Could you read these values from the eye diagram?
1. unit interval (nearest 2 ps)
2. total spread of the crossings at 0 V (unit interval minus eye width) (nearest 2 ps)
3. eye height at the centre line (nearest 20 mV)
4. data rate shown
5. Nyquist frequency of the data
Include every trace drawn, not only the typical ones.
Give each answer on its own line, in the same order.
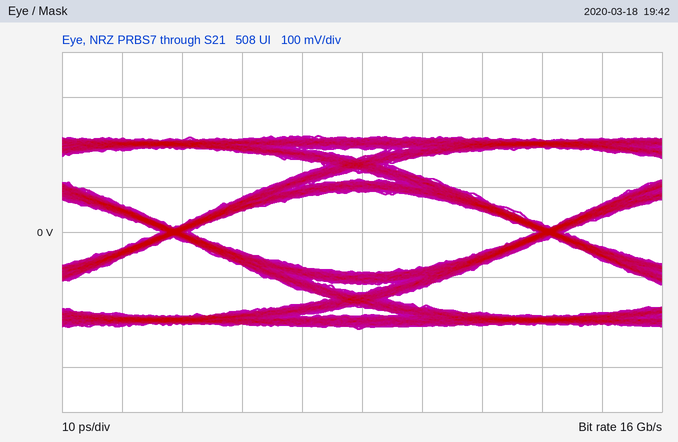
62 ps
4 ps
180 mV
16 Gb/s
8 GHz
